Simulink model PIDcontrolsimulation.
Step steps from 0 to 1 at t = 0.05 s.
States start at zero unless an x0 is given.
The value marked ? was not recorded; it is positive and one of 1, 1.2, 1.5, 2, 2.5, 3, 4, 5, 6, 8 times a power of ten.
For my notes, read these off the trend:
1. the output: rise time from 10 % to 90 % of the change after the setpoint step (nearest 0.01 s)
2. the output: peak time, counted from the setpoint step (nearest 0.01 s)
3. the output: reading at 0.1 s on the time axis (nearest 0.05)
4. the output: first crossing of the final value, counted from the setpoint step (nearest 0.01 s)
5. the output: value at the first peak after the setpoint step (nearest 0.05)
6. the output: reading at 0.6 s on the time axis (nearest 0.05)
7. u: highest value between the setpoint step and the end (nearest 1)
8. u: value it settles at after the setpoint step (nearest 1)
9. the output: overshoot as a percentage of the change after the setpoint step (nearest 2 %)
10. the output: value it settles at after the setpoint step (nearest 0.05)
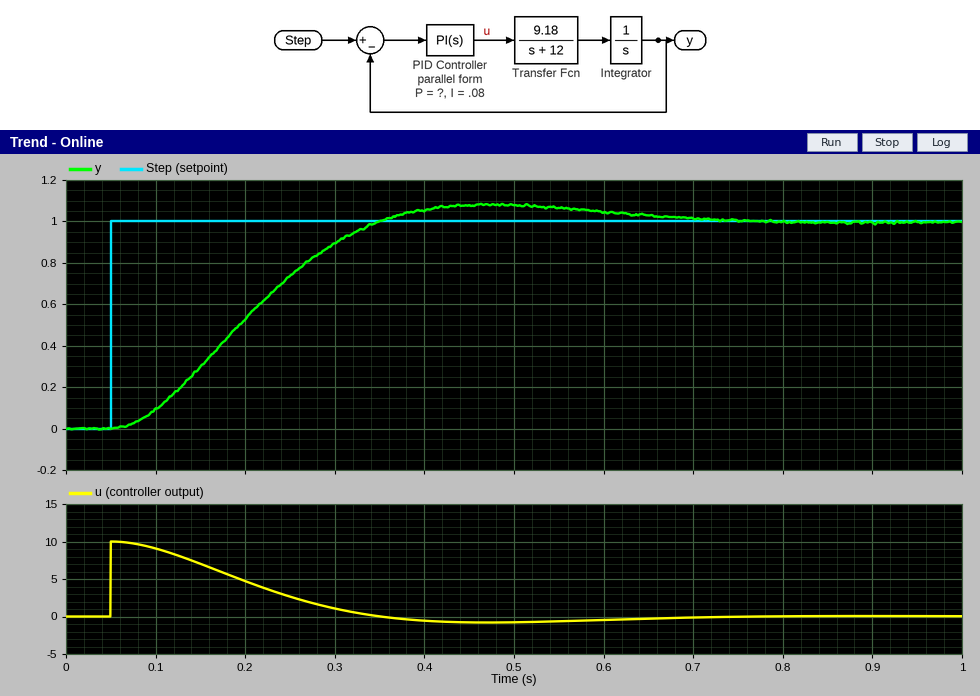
0.20 s
0.42 s
0.10
0.30 s
1.10
1.05
10
0
8 %
1.00
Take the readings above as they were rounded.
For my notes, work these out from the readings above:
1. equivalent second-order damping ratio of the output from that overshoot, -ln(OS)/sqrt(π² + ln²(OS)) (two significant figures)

0.63
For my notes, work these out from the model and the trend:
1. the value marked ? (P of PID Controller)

10
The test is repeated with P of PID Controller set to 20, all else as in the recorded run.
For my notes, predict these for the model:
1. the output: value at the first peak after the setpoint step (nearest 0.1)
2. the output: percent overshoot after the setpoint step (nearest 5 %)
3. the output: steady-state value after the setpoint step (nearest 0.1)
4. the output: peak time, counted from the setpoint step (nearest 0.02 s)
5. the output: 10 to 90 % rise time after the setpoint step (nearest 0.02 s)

1.2
20 %
1.0
0.26 s
0.12 s
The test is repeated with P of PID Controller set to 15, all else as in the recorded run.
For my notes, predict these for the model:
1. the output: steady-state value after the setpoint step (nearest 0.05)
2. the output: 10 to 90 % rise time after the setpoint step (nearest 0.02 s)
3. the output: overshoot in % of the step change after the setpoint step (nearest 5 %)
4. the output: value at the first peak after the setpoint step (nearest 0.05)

1.00
0.14 s
15 %
1.15
